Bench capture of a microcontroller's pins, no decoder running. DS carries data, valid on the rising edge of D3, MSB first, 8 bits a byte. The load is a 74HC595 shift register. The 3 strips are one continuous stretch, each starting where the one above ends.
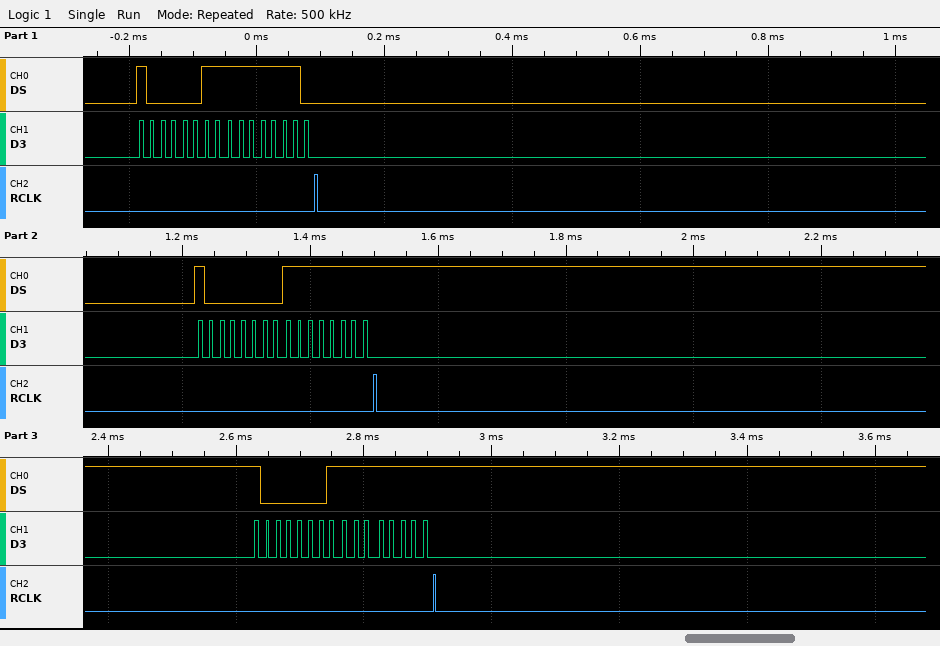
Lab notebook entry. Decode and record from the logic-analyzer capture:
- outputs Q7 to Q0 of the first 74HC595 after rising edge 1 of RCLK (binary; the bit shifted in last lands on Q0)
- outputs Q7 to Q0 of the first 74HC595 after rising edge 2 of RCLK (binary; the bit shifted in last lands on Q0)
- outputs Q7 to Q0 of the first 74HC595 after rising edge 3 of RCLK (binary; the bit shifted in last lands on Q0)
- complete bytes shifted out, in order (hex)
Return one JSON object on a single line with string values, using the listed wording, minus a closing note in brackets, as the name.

{"outputs Q7 to Q0 of the first 74HC595 after rising edge 1 of RCLK": "11111110", "outputs Q7 to Q0 of the first 74HC595 after rising edge 2 of RCLK": "11111111", "outputs Q7 to Q0 of the first 74HC595 after rising edge 3 of RCLK": "11111111", "complete bytes shifted out, in order": "0x83 0xFE 0x80 0xFF 0x81 0xFF"}
